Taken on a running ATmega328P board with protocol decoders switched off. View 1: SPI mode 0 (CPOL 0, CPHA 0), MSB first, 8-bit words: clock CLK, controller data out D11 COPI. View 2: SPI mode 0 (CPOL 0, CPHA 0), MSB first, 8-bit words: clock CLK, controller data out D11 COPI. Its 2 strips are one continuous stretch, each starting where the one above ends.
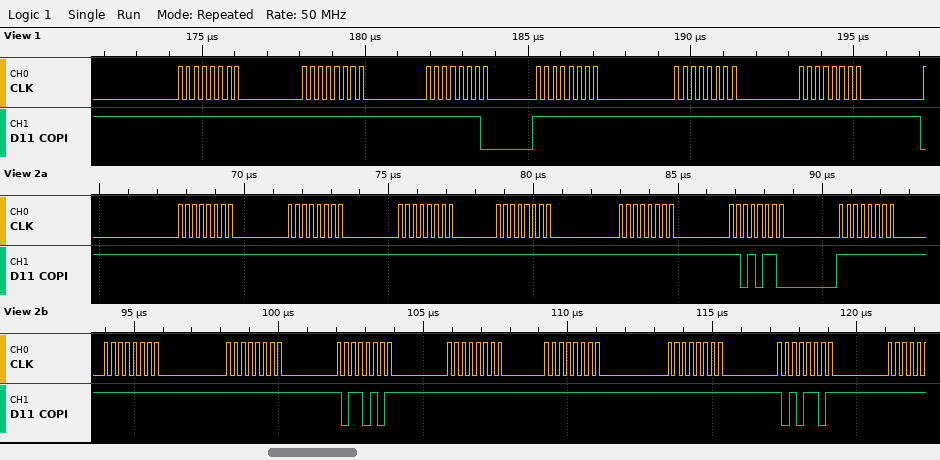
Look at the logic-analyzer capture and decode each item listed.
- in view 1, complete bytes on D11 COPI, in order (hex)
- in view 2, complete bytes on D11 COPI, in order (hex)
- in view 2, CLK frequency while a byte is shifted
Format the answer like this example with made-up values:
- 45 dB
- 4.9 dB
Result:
- FF FF FE FF FF FF
- 0xFF 0xFF 0xFF 0xFF 0xFF 0xD6 0xFF 0xFF 0xFF 0xB5 0xFF 0xFF 0xFF 0xAD
- 4 MHz
